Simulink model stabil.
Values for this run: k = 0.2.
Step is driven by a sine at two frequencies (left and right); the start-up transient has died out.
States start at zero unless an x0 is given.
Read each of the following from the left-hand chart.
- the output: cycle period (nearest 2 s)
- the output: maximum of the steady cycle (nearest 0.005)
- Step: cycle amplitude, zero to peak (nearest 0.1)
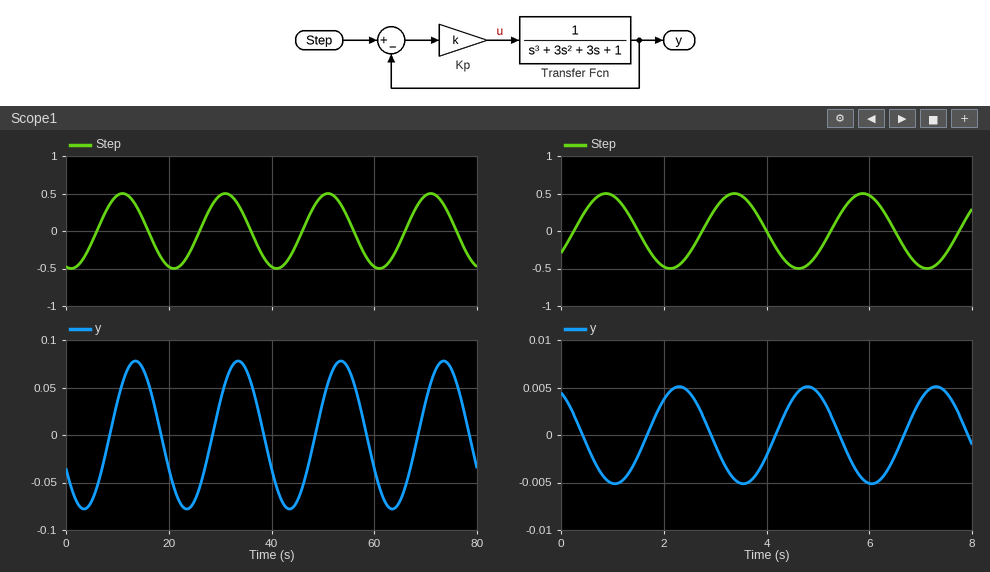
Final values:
20 s
0.080
0.5
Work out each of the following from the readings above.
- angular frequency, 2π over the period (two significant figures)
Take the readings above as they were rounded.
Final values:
0.31 rad/s
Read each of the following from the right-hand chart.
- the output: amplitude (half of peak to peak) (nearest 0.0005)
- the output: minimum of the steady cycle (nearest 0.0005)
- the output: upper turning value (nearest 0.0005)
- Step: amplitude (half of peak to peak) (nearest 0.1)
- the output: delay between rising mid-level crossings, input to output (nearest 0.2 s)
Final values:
0.0050
-0.0050
0.0050
0.5
1.4 s
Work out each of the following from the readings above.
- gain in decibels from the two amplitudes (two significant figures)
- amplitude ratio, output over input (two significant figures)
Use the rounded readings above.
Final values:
-40 dB
0.010
